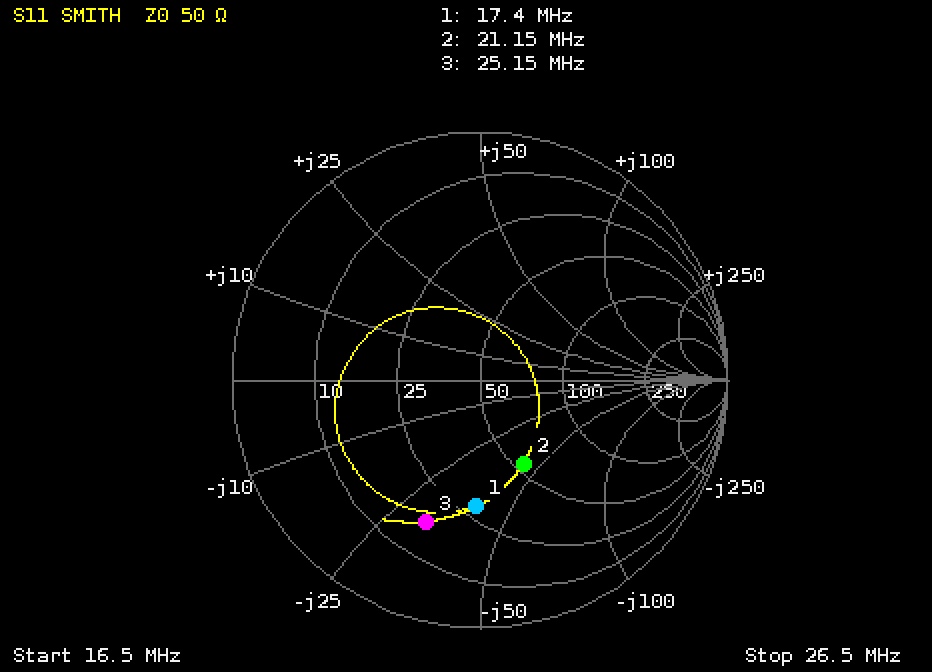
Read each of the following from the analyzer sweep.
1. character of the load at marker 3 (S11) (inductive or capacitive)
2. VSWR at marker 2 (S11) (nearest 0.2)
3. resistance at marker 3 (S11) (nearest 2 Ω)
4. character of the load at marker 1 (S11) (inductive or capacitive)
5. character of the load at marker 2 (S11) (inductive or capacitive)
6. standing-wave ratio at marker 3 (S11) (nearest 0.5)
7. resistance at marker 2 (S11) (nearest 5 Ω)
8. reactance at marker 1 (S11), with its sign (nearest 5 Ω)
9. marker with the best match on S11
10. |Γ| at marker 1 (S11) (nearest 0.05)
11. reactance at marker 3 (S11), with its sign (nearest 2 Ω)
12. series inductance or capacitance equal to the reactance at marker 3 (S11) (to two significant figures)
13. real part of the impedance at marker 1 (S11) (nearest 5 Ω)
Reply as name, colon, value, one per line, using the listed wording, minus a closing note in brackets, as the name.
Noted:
character of the load at marker 3 (S11): capacitive
VSWR at marker 2 (S11): 2.2
resistance at marker 3 (S11): 18 Ω
character of the load at marker 1 (S11): capacitive
character of the load at marker 2 (S11): capacitive
standing-wave ratio at marker 3 (S11): 4.0
resistance at marker 2 (S11): 55 Ω
reactance at marker 1 (S11), with its sign: -40 Ω
marker with the best match on S11: marker 2
|Γ| at marker 1 (S11): 0.50
reactance at marker 3 (S11), with its sign: -32 Ω
series inductance or capacitance equal to the reactance at marker 3 (S11): 200 pF
real part of the impedance at marker 1 (S11): 30 Ω
